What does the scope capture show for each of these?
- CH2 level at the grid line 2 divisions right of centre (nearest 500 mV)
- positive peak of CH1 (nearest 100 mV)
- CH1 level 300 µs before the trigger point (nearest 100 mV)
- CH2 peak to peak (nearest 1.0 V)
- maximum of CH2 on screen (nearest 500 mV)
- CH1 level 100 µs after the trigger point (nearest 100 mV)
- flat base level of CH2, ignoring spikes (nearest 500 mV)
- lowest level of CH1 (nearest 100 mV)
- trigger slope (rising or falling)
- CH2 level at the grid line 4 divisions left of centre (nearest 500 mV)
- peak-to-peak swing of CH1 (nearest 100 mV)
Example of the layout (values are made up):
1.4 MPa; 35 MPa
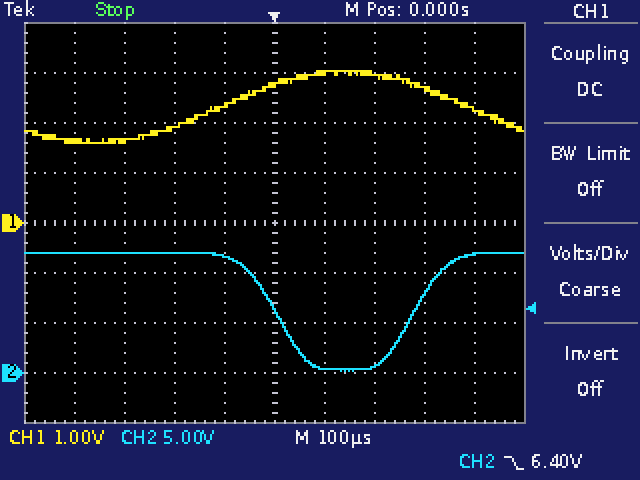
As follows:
500 mV; 3.0 V; 1.6 V; 12.0 V; 12.0 V; 3.0 V; 500 mV; 1.6 V; falling; 12.0 V; 1.4 V
